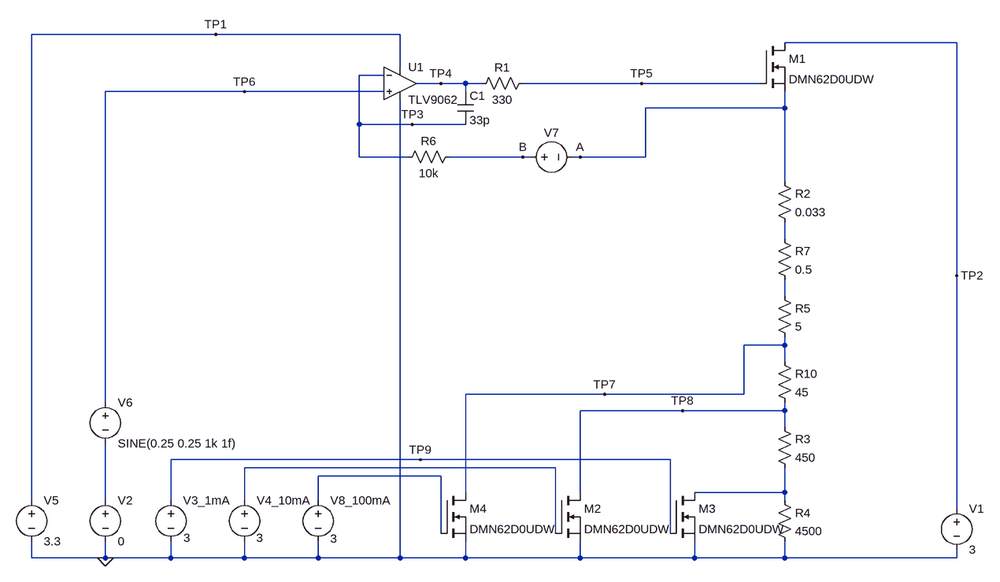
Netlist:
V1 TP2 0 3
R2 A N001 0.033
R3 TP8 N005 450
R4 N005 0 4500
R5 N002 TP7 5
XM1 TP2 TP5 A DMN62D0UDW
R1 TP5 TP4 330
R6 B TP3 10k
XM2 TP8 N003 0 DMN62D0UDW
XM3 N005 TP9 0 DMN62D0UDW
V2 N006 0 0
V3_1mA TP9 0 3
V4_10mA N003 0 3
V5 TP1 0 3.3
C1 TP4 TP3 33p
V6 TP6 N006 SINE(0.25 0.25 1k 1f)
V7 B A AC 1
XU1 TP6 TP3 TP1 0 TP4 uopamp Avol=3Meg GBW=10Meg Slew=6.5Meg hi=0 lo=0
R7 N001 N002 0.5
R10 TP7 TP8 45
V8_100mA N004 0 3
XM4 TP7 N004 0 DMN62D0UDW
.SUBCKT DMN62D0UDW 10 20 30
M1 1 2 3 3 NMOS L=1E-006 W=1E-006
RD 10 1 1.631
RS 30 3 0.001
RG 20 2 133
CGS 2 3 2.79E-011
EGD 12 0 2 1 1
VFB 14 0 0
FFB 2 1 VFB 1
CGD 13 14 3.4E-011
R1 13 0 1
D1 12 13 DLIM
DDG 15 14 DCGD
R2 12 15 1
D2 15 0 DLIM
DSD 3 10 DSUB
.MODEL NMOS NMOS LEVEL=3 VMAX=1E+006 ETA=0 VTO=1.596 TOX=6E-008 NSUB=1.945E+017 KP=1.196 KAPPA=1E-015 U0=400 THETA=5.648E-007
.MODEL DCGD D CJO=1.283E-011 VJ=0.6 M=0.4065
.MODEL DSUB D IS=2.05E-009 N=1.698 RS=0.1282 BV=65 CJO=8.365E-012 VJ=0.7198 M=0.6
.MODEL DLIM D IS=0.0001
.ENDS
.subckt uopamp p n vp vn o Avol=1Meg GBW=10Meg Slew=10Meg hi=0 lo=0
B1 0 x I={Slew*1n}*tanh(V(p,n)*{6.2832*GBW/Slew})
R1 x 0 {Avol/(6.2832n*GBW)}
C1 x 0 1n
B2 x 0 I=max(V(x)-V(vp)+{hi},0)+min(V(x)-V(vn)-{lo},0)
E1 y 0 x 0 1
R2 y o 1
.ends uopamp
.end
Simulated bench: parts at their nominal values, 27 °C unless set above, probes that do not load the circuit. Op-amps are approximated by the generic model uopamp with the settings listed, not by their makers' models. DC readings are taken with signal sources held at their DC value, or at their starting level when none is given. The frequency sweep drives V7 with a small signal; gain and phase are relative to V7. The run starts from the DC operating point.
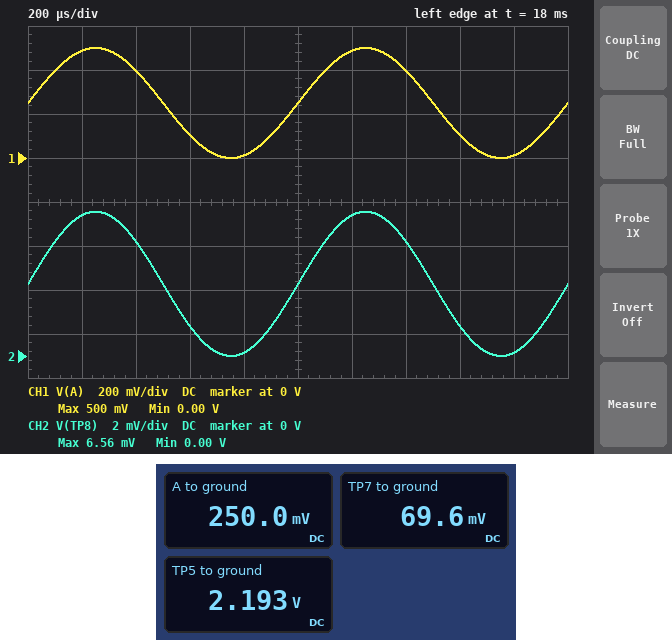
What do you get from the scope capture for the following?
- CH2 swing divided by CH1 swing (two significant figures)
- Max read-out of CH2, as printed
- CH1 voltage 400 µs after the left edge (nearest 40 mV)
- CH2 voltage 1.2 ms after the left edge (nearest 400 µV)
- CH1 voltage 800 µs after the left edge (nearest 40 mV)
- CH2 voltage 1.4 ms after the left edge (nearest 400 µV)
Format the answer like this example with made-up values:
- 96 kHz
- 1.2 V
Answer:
- 0.013
- 6.56 mV
- 400 mV
- 6.4 mV
- 0 V
- 5.2 mV
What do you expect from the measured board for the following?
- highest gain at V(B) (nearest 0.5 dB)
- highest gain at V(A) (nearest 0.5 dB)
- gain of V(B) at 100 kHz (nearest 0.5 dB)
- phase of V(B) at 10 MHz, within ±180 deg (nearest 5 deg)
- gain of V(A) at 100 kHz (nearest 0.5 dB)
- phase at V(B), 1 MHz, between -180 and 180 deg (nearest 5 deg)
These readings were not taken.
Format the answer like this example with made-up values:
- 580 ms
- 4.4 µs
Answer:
- 0.5 dB
- 0 dB
- -9.0 dB
- 0 deg
- -0.5 dB
- 15 deg
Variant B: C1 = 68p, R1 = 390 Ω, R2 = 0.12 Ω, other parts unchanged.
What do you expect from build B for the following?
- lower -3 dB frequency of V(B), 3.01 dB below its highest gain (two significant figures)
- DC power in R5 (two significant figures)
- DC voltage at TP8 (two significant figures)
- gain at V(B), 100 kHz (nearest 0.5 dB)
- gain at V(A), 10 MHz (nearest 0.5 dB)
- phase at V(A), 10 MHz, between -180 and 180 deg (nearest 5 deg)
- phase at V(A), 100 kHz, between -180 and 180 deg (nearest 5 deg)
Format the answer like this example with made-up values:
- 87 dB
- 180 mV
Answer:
- 140 kHz
- 5.2 mW
- 3.2 mV
- -4.5 dB
- -42.5 dB
- 10 deg
- 145 deg
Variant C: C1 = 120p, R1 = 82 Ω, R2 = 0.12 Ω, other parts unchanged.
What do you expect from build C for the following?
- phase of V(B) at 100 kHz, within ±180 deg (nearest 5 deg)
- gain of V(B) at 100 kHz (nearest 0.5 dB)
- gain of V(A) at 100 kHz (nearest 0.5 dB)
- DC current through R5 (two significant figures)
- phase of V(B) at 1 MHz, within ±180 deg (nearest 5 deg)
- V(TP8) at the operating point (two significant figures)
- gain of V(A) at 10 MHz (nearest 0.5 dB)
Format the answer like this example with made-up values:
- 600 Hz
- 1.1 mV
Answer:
- 40 deg
- -2.0 dB
- -4.0 dB
- 32 mA
- 5 deg
- 3.2 mV
- -46.0 dB
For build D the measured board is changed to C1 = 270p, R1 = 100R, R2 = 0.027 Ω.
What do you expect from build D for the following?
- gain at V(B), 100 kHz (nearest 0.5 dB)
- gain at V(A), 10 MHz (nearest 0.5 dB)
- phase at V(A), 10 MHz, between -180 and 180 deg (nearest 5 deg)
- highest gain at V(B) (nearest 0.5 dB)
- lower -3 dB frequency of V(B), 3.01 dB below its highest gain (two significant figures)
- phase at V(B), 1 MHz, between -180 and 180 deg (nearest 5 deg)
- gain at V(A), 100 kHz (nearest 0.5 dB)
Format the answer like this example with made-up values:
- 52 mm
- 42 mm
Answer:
- -0.5 dB
- -54.0 dB
- 30 deg
- 0 dB
- 35 kHz
- 0 deg
- -9.5 dB
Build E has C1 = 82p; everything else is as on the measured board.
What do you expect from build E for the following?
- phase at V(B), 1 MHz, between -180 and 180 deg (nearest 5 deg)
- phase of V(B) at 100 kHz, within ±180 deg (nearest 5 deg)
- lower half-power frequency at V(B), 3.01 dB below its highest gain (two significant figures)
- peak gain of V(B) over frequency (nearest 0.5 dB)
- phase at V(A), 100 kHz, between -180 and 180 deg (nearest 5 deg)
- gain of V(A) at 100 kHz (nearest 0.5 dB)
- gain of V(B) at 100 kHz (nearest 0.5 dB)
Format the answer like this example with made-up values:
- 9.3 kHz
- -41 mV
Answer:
- 5 deg
- 50 deg
- 110 kHz
- 0 dB
- 140 deg
- -2.5 dB
- -3.5 dB
